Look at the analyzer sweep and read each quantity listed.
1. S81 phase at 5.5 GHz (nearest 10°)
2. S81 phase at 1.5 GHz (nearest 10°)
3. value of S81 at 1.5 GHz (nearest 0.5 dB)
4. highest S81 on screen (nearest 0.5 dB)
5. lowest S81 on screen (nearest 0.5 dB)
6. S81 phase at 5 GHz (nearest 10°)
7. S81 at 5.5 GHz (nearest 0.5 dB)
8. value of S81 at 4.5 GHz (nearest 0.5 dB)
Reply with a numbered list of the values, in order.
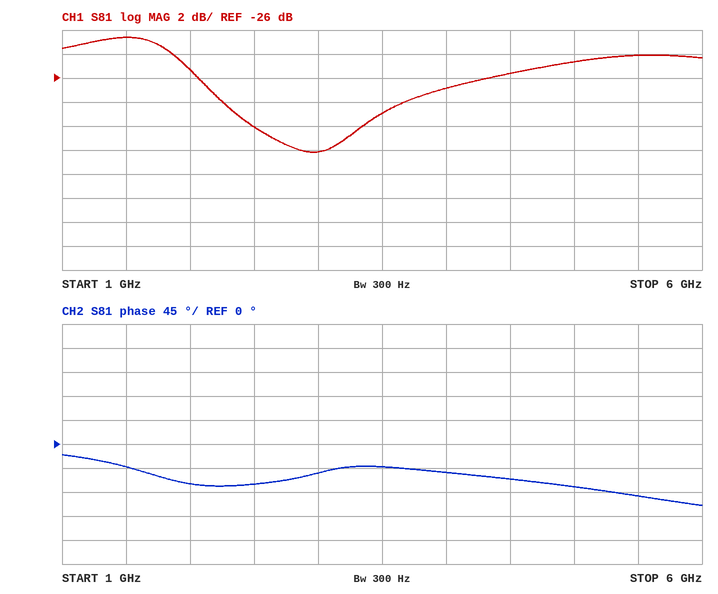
1. -100°
2. -40°
3. -22.5 dB
4. -22.5 dB
5. -32.0 dB
6. -80°
7. -24.0 dB
8. -25.5 dB
